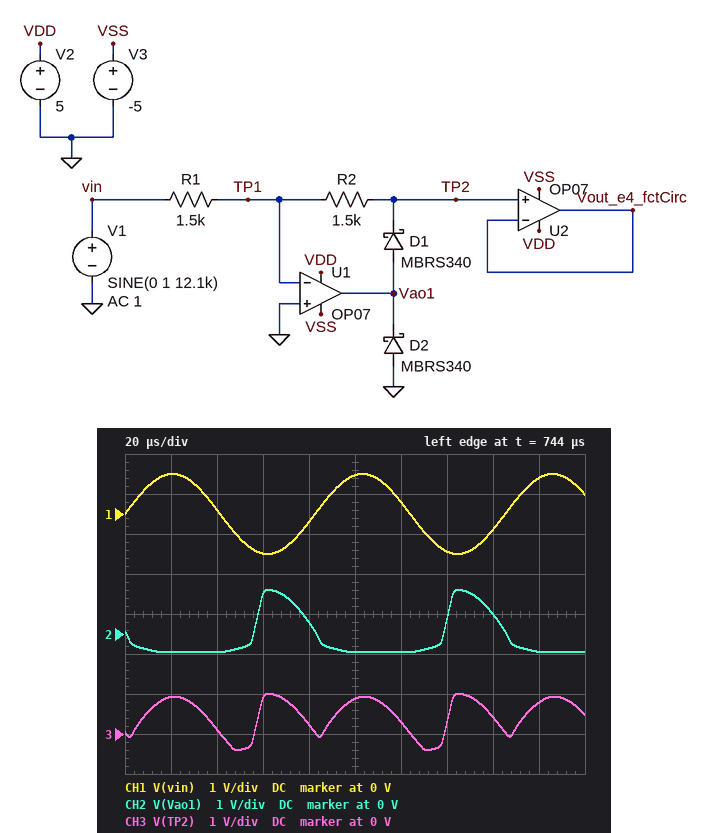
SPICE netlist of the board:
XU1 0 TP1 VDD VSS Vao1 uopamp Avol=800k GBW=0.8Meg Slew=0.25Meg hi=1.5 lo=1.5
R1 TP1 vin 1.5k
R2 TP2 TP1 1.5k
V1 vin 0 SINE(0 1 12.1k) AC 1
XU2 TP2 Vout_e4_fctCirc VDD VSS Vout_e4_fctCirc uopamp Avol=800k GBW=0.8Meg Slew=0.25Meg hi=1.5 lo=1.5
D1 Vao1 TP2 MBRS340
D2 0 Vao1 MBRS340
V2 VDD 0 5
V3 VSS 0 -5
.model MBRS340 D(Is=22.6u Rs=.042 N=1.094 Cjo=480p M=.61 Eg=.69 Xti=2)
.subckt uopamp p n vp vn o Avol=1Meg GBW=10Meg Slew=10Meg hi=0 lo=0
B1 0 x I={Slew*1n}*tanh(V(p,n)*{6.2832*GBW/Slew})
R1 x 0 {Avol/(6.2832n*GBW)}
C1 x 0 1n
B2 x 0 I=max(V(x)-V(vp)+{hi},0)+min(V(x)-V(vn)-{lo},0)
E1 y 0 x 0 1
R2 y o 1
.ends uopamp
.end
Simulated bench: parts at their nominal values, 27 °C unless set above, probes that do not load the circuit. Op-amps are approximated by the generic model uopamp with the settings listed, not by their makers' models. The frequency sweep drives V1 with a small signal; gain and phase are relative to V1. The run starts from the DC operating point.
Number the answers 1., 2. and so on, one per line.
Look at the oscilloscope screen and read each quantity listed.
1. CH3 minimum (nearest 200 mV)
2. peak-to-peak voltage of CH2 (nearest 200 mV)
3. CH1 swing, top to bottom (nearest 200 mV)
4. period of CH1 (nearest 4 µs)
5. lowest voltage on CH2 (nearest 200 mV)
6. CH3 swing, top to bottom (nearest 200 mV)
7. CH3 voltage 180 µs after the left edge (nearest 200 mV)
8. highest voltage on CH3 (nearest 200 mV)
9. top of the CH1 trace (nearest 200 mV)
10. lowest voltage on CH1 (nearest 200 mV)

1. -400 mV
2. 1.6 V
3. 2.0 V
4. 84 µs
5. -400 mV
6. 1.4 V
7. 800 mV
8. 1.0 V
9. 1.0 V
10. -1.0 V
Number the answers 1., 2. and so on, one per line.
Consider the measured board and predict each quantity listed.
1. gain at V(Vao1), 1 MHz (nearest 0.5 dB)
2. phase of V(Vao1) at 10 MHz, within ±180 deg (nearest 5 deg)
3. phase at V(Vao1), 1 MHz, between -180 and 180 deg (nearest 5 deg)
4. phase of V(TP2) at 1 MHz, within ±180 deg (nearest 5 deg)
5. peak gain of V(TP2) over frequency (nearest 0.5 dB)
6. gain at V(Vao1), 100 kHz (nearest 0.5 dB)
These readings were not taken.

1. -8.5 dB
2. 90 deg
3. 105 deg
4. 110 deg
5. 0 dB
6. 4.0 dB
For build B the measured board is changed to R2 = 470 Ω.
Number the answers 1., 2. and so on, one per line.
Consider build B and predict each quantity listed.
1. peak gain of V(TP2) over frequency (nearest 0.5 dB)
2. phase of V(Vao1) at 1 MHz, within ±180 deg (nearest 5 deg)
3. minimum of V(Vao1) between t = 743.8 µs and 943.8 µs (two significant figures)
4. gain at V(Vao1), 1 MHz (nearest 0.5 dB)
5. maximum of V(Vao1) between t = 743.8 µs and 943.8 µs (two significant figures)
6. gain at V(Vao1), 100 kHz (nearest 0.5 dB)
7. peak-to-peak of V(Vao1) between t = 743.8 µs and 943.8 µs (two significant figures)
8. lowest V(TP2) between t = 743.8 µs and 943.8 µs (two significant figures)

1. -10.0 dB
2. 95 deg
3. -460 mV
4. -14.0 dB
5. 410 mV
6. 0 dB
7. 870 mV
8. -410 mV
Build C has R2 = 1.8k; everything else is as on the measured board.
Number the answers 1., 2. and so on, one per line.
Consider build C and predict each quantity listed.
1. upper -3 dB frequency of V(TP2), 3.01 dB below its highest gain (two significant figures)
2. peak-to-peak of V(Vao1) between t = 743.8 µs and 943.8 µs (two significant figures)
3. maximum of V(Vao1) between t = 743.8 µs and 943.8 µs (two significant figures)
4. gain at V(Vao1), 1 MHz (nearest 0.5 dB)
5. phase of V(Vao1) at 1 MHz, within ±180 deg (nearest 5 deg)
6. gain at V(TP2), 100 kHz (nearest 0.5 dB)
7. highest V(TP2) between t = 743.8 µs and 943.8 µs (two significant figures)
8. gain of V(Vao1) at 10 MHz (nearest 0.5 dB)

1. 200 kHz
2. 1.8 V
3. 1.3 V
4. -7.5 dB
5. 105 deg
6. 0.5 dB
7. 1.2 V
8. -27.0 dB
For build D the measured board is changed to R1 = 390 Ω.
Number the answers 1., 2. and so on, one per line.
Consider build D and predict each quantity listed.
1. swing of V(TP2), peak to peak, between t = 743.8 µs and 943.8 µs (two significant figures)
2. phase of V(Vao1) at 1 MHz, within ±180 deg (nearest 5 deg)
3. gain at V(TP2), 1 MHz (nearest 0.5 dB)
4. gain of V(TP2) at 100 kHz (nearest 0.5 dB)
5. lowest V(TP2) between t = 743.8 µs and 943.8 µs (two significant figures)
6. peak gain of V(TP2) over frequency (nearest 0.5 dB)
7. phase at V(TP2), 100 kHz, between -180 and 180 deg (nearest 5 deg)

1. 3.6 V
2. 95 deg
3. -7.5 dB
4. 8.0 dB
5. -410 mV
6. 11.5 dB
7. 135 deg
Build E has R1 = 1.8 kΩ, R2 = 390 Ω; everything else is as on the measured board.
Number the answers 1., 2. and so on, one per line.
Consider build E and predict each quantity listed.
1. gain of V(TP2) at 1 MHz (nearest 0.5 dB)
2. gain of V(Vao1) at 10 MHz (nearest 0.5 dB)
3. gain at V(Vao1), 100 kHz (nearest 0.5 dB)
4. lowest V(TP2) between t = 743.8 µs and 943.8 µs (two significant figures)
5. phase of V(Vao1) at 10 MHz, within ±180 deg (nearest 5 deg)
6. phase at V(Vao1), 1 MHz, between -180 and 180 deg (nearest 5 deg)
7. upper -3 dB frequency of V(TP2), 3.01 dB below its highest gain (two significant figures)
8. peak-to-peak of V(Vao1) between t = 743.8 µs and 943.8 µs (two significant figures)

1. -30.5 dB
2. -37.0 dB
3. -2.0 dB
4. -410 mV
5. 85 deg
6. 95 deg
7. 190 kHz
8. 770 mV
